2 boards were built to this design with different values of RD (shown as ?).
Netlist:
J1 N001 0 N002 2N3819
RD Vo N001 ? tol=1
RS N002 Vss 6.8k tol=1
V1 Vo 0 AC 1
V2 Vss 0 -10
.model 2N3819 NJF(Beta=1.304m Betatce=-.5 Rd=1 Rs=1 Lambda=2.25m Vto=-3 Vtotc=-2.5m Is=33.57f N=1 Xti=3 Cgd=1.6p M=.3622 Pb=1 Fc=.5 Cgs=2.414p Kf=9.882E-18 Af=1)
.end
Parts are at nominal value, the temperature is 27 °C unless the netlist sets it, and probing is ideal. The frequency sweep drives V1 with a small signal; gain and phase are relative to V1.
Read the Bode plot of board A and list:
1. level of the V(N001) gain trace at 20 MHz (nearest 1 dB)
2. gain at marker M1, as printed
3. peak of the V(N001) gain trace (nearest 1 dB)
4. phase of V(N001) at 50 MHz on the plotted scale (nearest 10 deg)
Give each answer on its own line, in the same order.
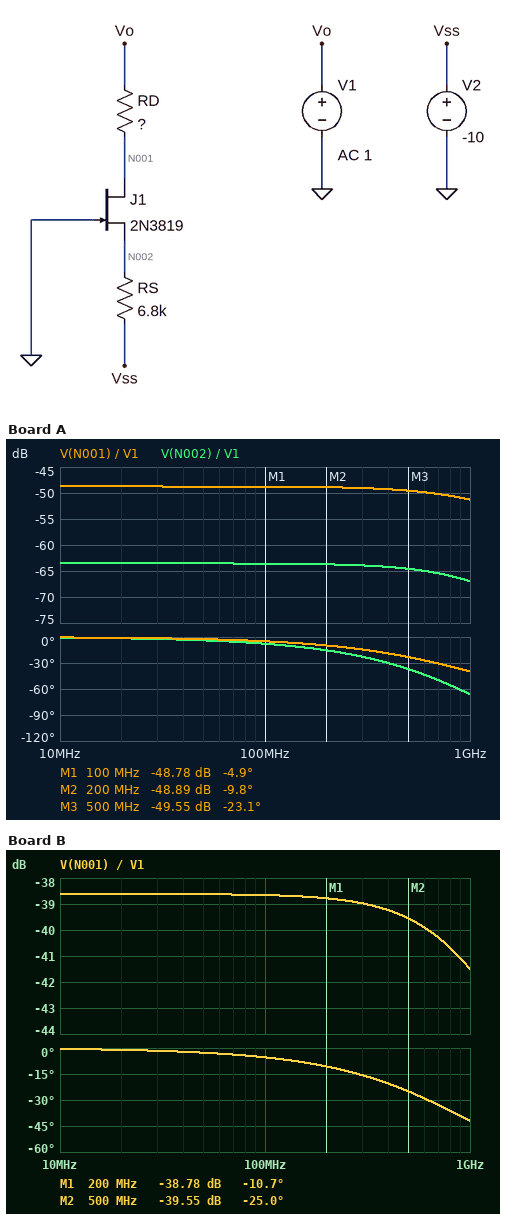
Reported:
-49 dB
-48.78 dB
-49 dB
0 deg
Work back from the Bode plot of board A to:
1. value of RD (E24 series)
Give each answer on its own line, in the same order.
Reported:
15 kΩ
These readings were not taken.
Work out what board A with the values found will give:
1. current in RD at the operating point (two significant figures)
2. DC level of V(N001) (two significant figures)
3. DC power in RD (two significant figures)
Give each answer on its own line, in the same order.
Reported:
39 µA
-590 mV
23 µW
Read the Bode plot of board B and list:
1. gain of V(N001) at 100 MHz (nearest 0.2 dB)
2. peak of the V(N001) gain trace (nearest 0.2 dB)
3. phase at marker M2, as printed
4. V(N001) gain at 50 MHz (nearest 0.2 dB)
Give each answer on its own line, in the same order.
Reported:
-38.6 dB
-38.6 dB
-25.0 deg
-38.6 dB
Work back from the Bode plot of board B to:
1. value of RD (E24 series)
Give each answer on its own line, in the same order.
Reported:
5.1 kΩ
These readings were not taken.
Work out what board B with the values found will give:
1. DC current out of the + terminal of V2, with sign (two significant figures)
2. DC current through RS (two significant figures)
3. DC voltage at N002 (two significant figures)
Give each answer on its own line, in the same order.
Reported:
-1.4 mA
1.4 mA
-630 mV
